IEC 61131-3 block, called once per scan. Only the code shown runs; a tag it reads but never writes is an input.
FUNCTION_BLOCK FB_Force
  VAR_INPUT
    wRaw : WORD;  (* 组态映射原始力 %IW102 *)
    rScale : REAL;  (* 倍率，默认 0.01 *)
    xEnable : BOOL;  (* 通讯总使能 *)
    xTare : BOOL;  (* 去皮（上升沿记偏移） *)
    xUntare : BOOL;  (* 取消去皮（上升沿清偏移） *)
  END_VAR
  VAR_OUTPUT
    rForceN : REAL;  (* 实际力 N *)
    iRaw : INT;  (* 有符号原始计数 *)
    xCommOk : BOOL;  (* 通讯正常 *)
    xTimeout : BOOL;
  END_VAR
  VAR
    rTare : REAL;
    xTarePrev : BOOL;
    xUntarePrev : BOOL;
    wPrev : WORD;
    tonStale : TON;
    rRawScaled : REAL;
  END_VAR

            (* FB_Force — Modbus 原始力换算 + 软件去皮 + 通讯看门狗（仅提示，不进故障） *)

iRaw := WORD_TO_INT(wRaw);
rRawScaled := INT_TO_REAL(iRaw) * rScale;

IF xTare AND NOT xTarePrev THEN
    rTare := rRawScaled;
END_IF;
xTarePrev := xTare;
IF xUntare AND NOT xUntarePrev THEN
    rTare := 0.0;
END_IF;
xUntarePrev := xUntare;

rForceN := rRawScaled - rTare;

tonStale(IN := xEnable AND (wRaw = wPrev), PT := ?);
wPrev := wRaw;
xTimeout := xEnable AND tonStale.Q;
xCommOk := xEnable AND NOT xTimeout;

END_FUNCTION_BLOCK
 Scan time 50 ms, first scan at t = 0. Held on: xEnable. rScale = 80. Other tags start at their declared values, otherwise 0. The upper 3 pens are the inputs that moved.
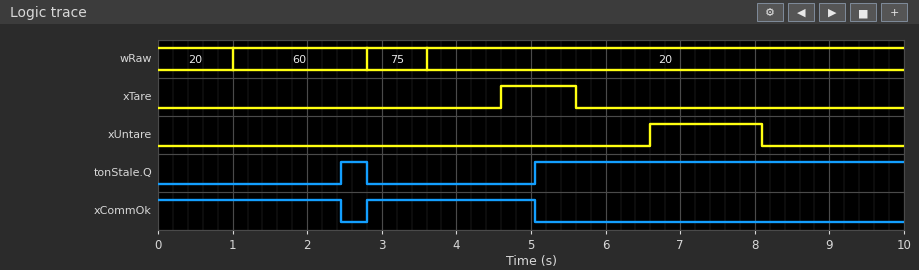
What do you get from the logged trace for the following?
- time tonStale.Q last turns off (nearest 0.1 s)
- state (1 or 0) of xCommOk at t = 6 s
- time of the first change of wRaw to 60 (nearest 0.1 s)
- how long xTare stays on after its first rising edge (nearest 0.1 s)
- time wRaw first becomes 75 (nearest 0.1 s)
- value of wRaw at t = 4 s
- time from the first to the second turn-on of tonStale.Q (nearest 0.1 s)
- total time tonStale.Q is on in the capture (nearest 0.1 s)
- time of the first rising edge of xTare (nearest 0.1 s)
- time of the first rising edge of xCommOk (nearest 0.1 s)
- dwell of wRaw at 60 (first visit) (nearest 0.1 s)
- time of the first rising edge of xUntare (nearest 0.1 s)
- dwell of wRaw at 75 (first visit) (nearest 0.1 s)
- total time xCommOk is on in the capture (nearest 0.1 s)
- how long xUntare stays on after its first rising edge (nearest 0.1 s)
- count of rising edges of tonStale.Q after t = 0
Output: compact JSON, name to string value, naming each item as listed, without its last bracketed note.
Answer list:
{"time tonStale.Q last turns off": "2.8 s", "state (1 or 0) of xCommOk at t = 6 s": "0", "time of the first change of wRaw to 60": "1.0 s", "how long xTare stays on after its first rising edge": "1.0 s", "time wRaw first becomes 75": "2.8 s", "value of wRaw at t = 4 s": "20", "time from the first to the second turn-on of tonStale.Q": "2.6 s", "total time tonStale.Q is on in the capture": "5.3 s", "time of the first rising edge of xTare": "4.6 s", "time of the first rising edge of xCommOk": "2.8 s", "dwell of wRaw at 60 (first visit)": "1.8 s", "time of the first rising edge of xUntare": "6.6 s", "dwell of wRaw at 75 (first visit)": "0.8 s", "total time xCommOk is on in the capture": "4.7 s", "how long xUntare stays on after its first rising edge": "1.5 s", "count of rising edges of tonStale.Q after t = 0": "2"}
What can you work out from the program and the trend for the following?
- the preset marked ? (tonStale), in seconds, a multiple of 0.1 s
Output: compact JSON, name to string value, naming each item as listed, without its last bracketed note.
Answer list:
{"the preset marked ? (tonStale), in seconds, a multiple of 0.1 s": "1.4 s"}
